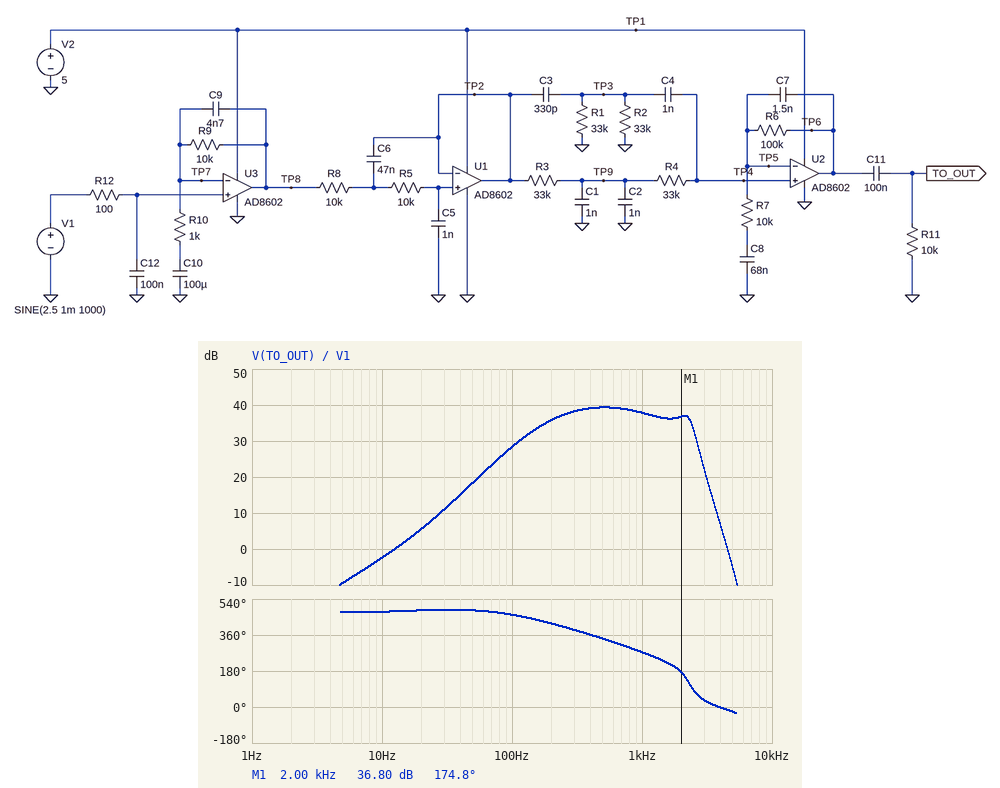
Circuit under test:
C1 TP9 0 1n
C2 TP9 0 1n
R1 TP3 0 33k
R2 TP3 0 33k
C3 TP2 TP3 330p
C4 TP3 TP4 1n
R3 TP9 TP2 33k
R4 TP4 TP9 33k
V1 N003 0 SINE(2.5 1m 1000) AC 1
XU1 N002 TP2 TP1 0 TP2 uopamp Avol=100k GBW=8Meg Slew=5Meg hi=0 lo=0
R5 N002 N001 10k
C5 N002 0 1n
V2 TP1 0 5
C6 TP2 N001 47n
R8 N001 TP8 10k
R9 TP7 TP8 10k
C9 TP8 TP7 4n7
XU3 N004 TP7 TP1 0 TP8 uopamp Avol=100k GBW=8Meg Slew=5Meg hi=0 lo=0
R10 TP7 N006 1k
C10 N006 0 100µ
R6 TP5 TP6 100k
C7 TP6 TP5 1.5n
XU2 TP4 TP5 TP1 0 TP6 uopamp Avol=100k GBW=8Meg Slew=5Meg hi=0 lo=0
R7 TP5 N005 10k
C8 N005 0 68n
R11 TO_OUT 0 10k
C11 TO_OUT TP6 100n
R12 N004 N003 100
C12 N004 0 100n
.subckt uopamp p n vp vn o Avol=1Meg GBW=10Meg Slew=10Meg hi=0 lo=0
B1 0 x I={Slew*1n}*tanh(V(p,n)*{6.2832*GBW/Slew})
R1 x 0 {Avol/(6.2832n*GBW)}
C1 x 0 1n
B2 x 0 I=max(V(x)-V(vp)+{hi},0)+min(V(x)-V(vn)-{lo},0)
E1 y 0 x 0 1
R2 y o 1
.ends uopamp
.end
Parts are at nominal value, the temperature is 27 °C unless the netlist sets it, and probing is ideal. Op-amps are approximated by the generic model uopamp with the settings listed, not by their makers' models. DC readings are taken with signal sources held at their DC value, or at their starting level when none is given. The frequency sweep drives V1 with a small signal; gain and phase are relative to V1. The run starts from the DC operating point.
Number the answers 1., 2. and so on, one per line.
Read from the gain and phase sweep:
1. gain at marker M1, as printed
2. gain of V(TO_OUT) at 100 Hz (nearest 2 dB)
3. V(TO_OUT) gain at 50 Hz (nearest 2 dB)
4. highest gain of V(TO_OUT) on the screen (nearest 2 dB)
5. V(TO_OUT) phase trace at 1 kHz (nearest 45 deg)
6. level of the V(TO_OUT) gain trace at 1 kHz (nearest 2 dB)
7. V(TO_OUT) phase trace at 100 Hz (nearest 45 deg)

1. 36.80 dB
2. 28 dB
3. 18 dB
4. 40 dB
5. 270 deg
6. 38 dB
7. 450 deg
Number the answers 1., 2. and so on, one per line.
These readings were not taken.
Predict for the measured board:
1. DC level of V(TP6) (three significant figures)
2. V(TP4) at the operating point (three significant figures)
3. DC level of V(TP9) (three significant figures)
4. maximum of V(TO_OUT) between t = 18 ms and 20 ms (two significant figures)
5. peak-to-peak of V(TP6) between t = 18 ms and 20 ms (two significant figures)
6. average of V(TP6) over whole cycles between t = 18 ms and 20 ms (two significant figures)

1. 2.50 V
2. 2.50 V
3. 2.50 V
4. 78 mV
5. 160 mV
6. 2.5 V
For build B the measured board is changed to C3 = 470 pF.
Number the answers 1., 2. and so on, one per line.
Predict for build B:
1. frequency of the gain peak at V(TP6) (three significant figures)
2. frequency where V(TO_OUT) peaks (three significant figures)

1. 449 Hz
2. 511 Hz
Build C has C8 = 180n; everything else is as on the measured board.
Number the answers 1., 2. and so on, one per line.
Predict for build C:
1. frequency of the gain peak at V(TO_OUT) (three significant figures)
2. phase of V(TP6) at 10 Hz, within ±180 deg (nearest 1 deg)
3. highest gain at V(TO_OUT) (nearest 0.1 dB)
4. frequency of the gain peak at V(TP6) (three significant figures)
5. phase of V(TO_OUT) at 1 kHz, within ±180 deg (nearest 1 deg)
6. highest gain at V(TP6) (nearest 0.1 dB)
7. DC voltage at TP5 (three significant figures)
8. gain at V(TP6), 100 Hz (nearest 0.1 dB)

1. 407 Hz
2. 52 deg
3. 40.1 dB
4. 279 Hz
5. -93 deg
6. 40.9 dB
7. 2.50 V
8. 39.2 dB
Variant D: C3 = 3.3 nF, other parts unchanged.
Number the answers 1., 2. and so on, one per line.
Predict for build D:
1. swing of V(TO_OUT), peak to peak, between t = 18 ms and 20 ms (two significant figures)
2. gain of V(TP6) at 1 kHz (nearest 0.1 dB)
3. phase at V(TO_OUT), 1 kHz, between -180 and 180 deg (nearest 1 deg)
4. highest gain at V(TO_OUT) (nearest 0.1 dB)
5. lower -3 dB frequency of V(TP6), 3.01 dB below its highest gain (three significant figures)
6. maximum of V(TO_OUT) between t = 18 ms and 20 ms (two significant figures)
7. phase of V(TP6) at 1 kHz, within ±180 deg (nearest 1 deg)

1. 140 mV
2. 37.0 dB
3. -84 deg
4. 39.1 dB
5. 155 Hz
6. 70 mV
7. -93 deg
